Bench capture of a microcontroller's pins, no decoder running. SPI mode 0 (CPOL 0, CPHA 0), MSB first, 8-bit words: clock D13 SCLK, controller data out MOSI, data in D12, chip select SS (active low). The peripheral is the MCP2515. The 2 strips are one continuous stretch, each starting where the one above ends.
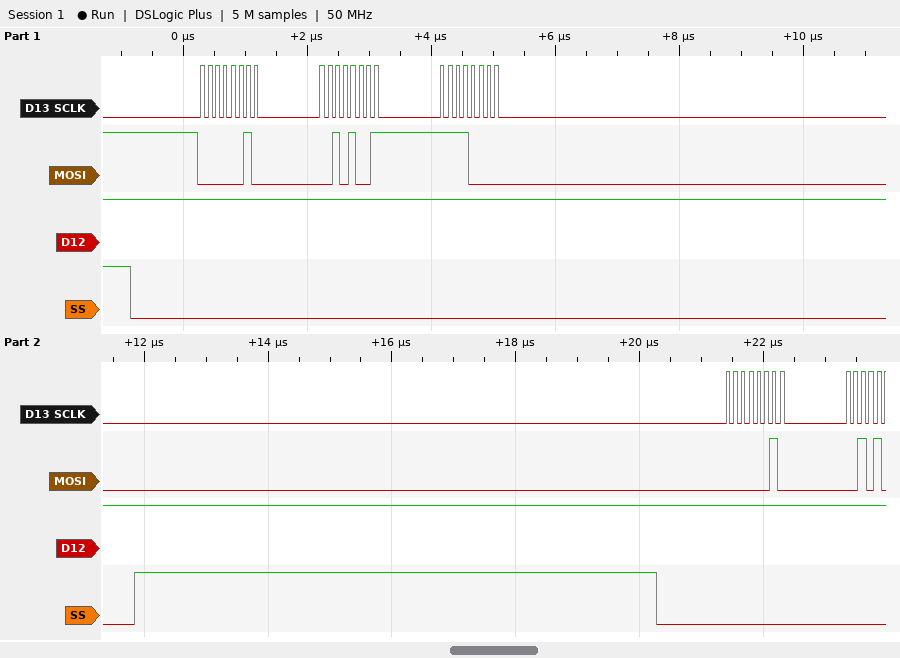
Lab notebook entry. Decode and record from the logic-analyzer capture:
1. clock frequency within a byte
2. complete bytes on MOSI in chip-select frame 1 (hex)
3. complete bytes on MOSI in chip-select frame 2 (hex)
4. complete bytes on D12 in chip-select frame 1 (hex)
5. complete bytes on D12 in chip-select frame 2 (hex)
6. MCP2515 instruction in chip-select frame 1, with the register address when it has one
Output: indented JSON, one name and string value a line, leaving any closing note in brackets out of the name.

{
  "clock frequency within a byte": "8 MHz",
  "complete bytes on MOSI in chip-select frame 1": "02 29 F0",
  "complete bytes on MOSI in chip-select frame 2": "02",
  "complete bytes on D12 in chip-select frame 1": "FF FF FF",
  "complete bytes on D12 in chip-select frame 2": "FF",
  "MCP2515 instruction in chip-select frame 1, with the register address when it has one": "WRITE 0x29"
}
